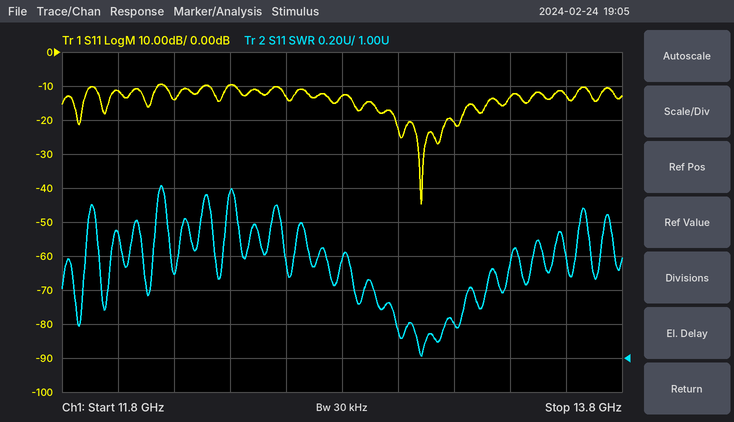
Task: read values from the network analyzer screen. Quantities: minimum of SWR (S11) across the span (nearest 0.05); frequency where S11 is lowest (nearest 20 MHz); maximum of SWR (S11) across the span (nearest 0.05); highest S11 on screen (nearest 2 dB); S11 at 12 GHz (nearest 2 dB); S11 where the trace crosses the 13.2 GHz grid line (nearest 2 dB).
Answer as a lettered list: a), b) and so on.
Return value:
a) 1.00
b) 13.08 GHz
c) 2.00
d) -10 dB
e) -12 dB
f) -20 dB
